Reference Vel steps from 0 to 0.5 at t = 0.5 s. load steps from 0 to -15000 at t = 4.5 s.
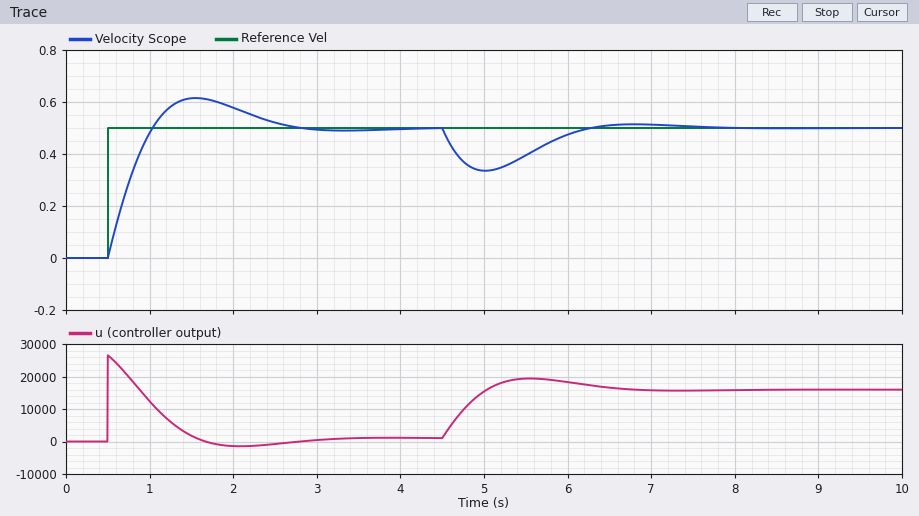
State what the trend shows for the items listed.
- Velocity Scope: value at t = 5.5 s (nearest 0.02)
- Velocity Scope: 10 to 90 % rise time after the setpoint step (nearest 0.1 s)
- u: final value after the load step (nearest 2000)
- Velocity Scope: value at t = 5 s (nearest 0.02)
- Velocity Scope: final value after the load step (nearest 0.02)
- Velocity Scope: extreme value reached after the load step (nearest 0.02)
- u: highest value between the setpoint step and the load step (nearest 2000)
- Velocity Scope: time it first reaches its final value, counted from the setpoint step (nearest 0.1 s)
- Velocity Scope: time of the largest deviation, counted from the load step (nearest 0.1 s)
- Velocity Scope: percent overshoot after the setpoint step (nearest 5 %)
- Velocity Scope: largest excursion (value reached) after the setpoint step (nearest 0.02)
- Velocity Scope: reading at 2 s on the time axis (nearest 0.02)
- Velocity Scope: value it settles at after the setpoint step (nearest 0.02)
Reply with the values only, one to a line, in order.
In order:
0.40
0.4 s
16000
0.34
0.50
0.34
26000
0.5 s
0.5 s
25 %
0.62
0.58
0.50
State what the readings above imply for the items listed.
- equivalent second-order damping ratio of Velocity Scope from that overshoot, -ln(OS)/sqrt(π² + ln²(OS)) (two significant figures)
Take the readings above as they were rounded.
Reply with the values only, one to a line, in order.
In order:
0.40
